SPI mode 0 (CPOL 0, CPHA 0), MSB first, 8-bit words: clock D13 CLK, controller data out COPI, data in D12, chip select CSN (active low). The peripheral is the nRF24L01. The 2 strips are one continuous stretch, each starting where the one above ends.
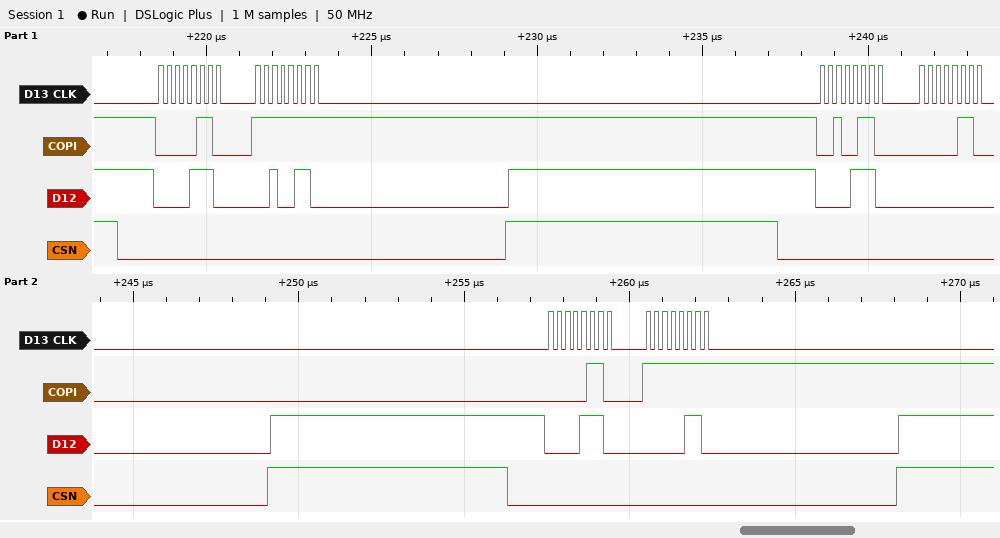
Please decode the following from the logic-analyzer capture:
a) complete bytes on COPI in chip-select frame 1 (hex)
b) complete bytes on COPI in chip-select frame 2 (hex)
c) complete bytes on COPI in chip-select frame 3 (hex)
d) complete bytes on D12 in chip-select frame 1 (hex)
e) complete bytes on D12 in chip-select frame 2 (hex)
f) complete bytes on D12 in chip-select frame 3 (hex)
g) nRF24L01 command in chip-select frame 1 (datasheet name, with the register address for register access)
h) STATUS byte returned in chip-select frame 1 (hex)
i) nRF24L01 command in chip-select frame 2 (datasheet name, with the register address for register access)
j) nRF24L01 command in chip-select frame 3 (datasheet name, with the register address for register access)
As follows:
0x06 0xFF
0x26 0x06
0x06 0xFF
0x0E 0x26
0x0E 0x00
0x0E 0x06
R_REGISTER 0x06
0x0E
W_REGISTER 0x06
R_REGISTER 0x06
